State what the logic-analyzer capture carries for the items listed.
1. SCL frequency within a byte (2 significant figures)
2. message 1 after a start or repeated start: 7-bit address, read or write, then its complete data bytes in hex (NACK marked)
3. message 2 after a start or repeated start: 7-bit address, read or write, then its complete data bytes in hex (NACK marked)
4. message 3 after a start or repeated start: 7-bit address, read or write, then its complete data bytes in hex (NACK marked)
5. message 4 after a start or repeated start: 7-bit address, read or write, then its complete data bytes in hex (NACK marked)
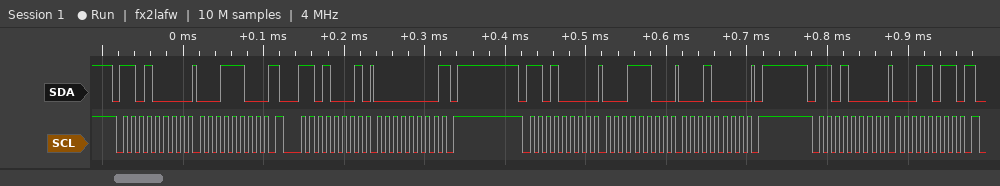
100 kHz
0x68 write: 1C
0x68 read: 00 NACK
0x68 write: 1C 10
0x68 write: 1B
